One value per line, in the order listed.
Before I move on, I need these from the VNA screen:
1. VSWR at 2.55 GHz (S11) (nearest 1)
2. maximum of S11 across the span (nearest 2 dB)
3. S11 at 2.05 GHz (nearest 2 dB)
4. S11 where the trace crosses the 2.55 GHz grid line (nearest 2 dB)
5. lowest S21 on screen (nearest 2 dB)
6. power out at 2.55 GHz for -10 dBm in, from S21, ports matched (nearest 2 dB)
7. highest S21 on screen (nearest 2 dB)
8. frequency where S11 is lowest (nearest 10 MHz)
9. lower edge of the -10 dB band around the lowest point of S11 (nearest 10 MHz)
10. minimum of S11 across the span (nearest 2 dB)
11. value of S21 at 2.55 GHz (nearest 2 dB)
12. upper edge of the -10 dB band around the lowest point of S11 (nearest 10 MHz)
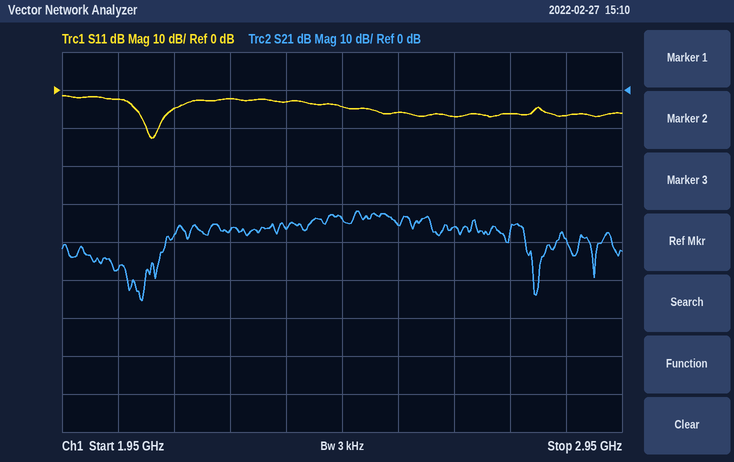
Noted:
3
-2 dB
-2 dB
-6 dB
-56 dB
-46 dBm
-32 dB
2.11 GHz
2.10 GHz
-12 dB
-36 dB
2.12 GHz
